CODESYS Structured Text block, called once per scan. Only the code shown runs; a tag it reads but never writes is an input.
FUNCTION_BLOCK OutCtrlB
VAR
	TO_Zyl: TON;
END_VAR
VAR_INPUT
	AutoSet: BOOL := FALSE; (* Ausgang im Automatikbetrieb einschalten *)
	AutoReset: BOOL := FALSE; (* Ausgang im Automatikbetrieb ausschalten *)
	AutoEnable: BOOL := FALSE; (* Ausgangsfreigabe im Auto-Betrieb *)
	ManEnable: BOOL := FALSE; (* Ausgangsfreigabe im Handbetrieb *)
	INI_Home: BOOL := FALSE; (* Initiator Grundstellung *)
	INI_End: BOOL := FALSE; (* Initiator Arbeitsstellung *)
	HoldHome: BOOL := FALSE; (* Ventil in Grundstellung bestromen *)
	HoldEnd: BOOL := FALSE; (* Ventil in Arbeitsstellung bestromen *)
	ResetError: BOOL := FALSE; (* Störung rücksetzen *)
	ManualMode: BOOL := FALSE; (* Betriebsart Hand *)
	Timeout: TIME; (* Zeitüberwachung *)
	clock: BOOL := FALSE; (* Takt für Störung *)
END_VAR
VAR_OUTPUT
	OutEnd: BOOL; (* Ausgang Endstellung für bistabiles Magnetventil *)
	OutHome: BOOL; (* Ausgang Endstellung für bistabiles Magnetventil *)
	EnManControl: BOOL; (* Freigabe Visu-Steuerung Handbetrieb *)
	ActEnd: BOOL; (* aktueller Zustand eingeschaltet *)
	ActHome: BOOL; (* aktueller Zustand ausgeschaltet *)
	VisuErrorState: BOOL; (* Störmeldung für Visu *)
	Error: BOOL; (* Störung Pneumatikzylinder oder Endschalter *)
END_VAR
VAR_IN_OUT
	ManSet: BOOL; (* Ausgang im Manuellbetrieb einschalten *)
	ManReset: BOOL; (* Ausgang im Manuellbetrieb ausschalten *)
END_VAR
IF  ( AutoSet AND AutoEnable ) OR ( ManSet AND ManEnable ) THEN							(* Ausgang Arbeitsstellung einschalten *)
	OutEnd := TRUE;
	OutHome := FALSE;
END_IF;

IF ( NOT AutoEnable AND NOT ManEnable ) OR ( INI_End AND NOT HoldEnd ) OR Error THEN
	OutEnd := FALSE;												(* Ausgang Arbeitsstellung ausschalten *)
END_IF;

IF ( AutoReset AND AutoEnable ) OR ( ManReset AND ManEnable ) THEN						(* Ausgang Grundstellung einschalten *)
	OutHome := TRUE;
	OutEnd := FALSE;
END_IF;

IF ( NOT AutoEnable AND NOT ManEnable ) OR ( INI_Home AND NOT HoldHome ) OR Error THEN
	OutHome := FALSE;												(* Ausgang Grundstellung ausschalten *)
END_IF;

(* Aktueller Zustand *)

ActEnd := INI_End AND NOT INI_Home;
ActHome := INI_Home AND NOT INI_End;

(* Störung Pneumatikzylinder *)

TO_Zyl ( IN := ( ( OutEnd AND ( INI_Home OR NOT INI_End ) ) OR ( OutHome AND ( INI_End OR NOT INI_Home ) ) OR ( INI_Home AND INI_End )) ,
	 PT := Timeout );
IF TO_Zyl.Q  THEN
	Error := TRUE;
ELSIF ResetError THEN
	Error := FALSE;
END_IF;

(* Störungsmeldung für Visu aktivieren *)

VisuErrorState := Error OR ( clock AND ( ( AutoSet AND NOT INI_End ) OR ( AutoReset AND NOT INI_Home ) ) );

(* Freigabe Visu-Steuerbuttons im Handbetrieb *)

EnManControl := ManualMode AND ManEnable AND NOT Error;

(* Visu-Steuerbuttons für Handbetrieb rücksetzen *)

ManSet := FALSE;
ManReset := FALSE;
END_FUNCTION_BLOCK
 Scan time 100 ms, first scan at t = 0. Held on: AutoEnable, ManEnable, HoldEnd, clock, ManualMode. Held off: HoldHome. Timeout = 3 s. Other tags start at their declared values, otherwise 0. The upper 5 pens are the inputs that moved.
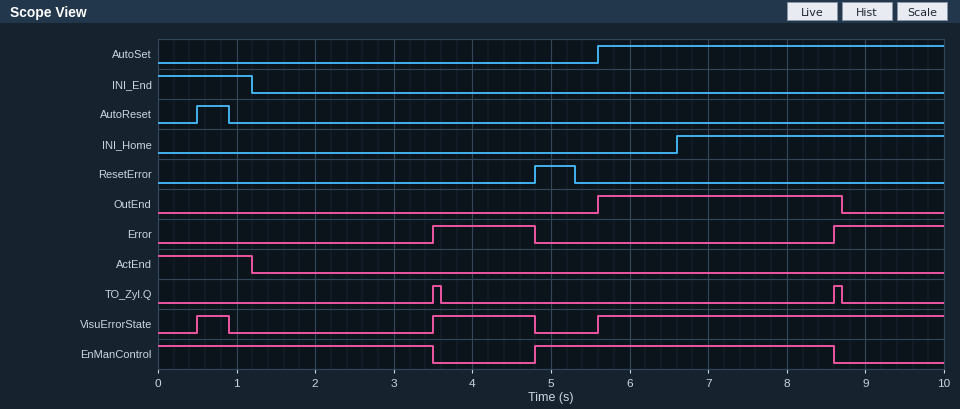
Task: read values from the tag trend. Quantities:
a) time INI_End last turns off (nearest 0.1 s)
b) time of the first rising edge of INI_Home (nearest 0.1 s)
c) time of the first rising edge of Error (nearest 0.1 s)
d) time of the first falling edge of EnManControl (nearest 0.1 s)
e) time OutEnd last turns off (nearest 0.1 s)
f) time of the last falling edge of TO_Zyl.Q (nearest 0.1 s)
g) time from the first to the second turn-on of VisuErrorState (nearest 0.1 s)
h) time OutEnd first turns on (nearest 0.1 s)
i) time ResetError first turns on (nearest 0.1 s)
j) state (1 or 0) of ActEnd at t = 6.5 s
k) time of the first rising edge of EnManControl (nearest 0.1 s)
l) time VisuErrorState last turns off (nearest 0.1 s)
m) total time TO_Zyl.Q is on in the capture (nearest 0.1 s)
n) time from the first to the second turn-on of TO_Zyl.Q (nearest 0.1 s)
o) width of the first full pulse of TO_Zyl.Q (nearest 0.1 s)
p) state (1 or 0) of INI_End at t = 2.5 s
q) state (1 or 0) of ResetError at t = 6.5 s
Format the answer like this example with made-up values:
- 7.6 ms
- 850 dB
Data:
- 1.2 s
- 6.6 s
- 3.5 s
- 3.5 s
- 8.7 s
- 8.7 s
- 3.0 s
- 5.6 s
- 4.8 s
- 0
- 4.8 s
- 4.8 s
- 0.2 s
- 5.1 s
- 0.1 s
- 0
- 0
